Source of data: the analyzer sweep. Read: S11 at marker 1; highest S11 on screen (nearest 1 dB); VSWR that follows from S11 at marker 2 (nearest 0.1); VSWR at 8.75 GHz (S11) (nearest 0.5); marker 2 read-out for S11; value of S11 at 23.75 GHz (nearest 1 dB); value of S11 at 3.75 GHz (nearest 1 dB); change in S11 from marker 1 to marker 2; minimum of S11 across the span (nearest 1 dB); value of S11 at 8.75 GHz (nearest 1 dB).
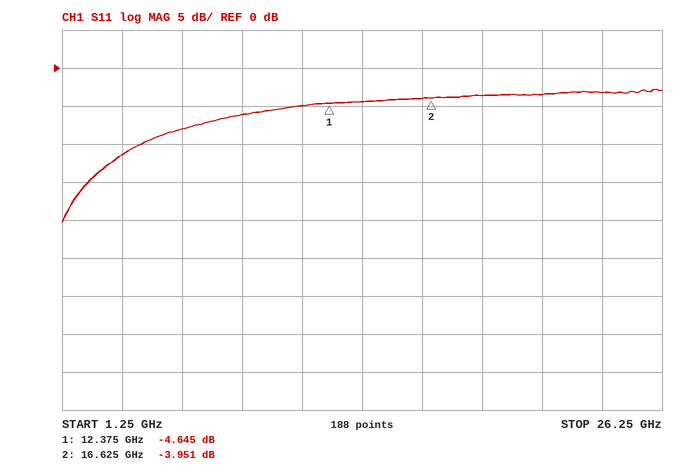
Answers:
-4.645 dB
-3 dB
4.5
3.0
-3.951 dB
-3 dB
-11 dB
0.694 dB
-20 dB
-6 dB
